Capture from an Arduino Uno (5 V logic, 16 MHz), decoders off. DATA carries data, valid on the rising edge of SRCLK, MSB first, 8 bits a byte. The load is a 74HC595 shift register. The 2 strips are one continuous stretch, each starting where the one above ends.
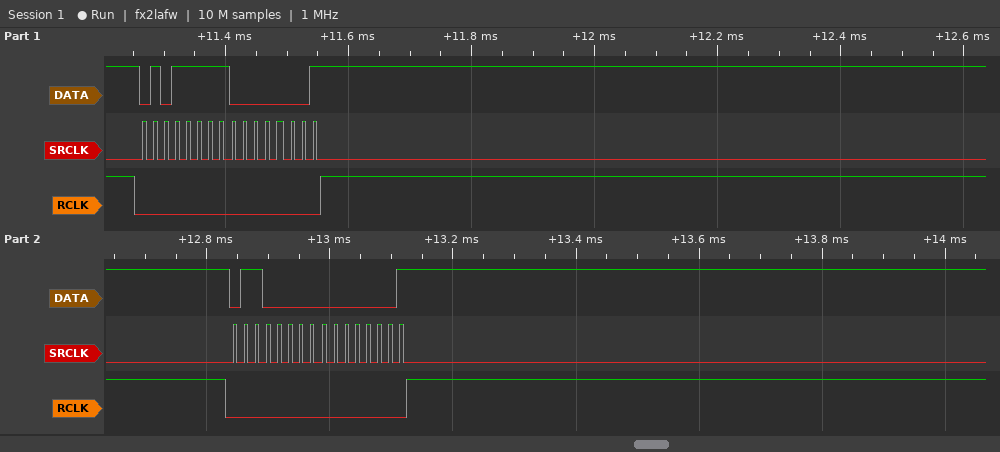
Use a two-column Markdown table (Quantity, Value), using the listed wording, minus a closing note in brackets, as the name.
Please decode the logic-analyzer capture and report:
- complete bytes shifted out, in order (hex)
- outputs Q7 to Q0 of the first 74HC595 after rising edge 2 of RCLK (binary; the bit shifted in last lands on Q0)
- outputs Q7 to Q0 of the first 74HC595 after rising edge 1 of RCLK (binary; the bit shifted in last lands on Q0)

| Quantity | Value |
|---|---|
| complete bytes shifted out, in order | 5F 01 60 01 |
| outputs Q7 to Q0 of the first 74HC595 after rising edge 2 of RCLK | 00000001 |
| outputs Q7 to Q0 of the first 74HC595 after rising edge 1 of RCLK | 00000001 |
